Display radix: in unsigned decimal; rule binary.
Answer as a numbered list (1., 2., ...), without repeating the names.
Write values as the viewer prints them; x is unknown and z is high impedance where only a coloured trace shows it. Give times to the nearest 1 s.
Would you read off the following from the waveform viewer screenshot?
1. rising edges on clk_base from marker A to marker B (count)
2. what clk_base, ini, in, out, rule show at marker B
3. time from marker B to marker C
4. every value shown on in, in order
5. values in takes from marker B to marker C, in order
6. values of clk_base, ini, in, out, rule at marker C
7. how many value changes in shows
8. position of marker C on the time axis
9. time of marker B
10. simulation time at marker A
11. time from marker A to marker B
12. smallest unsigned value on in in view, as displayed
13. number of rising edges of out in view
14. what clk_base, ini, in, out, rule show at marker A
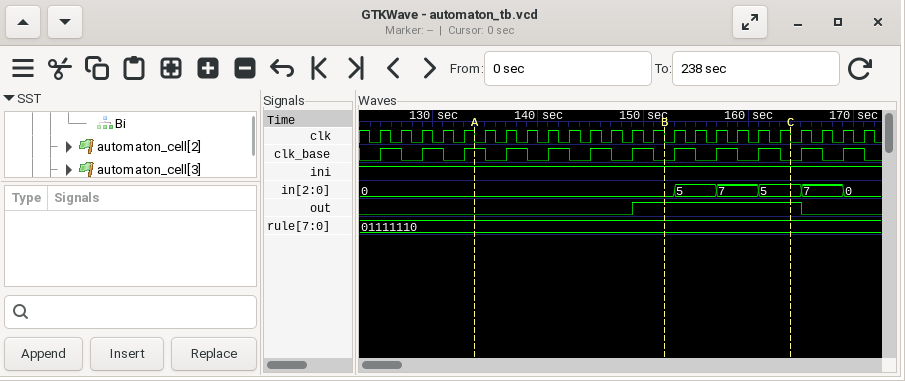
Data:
1. 4
2. clk_base=0, ini=1, in=0, out=1, rule=01111110
3. 12 s
4. 0, 5, 7, 5, 7, 0
5. 0, 5, 7, 5
6. clk_base=0, ini=1, in=5, out=1, rule=01111110
7. 5
8. 164 s
9. 152 s
10. 134 s
11. 18 s
12. 0
13. 1
14. clk_base=1, ini=1, in=0, out=0, rule=01111110
